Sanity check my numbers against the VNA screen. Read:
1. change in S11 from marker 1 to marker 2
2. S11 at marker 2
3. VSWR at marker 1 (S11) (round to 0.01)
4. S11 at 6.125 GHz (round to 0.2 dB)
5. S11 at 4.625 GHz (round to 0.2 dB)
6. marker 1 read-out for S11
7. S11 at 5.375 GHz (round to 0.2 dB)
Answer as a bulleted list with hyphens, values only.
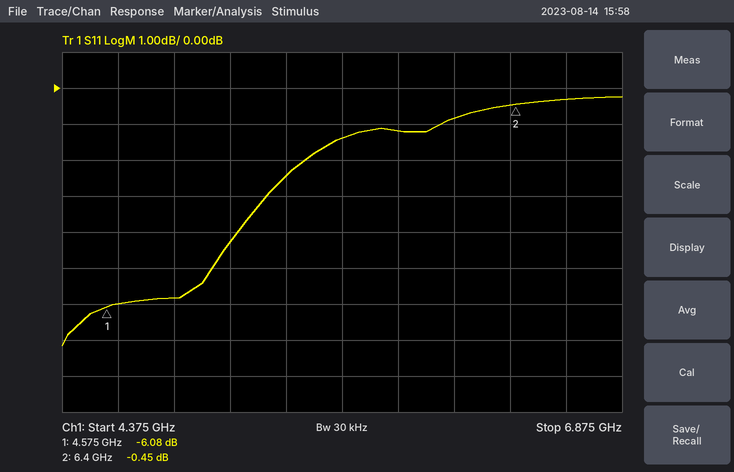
- 5.63 dB
- -0.45 dB
- 2.97
- -0.8 dB
- -6.0 dB
- -6.08 dB
- -2.4 dB
